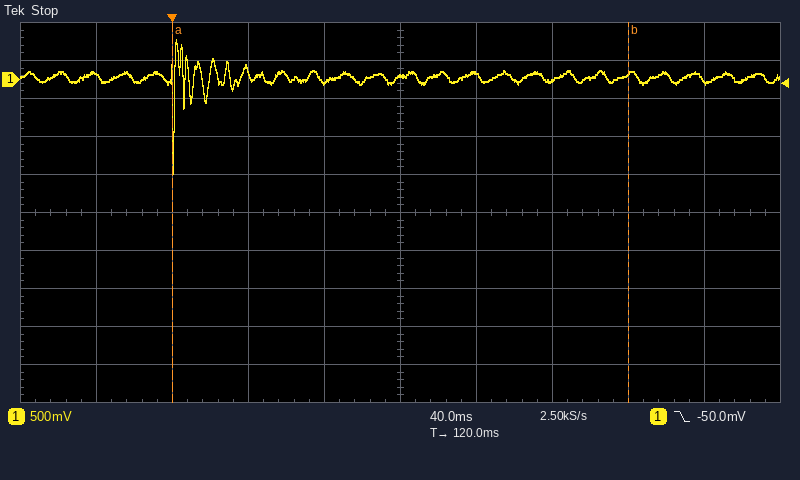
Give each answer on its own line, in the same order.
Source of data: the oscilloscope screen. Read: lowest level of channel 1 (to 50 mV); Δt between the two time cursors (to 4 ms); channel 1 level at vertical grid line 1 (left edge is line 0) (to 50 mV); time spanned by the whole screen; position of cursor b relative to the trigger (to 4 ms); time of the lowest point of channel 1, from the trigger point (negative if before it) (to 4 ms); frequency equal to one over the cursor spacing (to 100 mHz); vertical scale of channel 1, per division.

-1.25 V
240 ms
50 mV
400 ms
+240 ms
0 ms
4.2 Hz
500 mV
